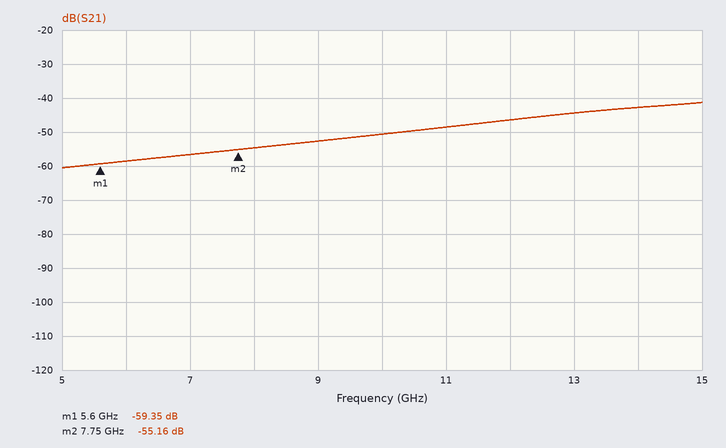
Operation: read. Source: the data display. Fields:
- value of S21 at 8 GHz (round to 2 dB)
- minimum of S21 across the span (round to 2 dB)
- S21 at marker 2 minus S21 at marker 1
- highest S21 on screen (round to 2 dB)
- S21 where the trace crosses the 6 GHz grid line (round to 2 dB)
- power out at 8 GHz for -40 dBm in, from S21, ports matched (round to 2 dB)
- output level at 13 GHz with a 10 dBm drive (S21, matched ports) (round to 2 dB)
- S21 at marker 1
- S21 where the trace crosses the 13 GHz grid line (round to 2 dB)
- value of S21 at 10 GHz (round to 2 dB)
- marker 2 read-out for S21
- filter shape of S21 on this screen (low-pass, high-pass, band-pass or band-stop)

-54 dB
-60 dB
4.19 dB
-42 dB
-58 dB
-94 dBm
-34 dBm
-59.35 dB
-44 dB
-50 dB
-55.16 dB
high-pass
